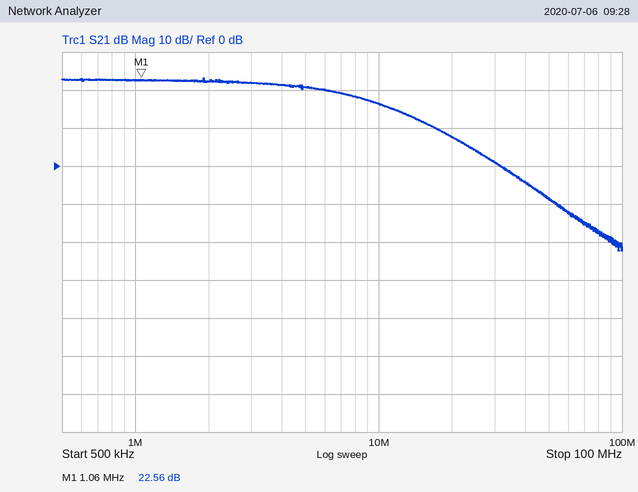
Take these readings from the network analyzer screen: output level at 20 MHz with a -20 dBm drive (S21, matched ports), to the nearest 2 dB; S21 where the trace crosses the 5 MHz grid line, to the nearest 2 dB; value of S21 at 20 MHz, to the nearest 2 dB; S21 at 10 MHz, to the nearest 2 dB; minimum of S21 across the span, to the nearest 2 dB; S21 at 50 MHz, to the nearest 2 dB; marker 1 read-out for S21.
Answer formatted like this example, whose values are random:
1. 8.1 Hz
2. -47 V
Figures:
1. -12 dBm
2. 20 dB
3. 8 dB
4. 16 dB
5. -22 dB
6. -8 dB
7. 22.56 dB
